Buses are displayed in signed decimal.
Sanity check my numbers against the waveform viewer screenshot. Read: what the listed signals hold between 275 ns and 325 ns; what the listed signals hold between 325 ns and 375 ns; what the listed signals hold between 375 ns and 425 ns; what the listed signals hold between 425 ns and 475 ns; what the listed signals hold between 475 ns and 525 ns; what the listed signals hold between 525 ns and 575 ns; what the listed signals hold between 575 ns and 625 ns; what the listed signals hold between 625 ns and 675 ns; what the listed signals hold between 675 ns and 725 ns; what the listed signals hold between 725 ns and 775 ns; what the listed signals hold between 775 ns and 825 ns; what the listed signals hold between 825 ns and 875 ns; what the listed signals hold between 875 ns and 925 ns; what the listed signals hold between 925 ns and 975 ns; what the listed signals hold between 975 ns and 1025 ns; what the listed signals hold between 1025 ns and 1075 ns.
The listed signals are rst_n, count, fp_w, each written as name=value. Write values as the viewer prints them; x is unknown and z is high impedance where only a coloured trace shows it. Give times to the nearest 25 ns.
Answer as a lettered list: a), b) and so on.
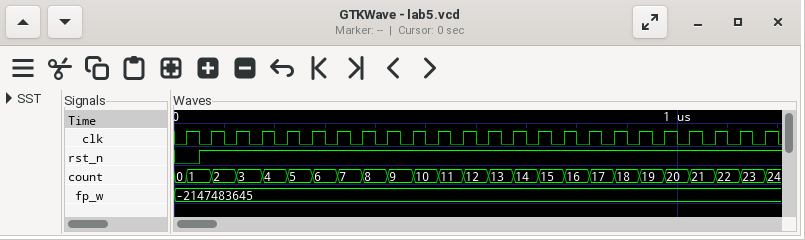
a) rst_n=1, count=6, fp_w=-2147483645
b) rst_n=1, count=7, fp_w=-2147483645
c) rst_n=1, count=8, fp_w=-2147483645
d) rst_n=1, count=9, fp_w=-2147483645
e) rst_n=1, count=10, fp_w=-2147483645
f) rst_n=1, count=11, fp_w=-2147483645
g) rst_n=1, count=12, fp_w=-2147483645
h) rst_n=1, count=13, fp_w=-2147483645
i) rst_n=1, count=14, fp_w=-2147483645
j) rst_n=1, count=15, fp_w=-2147483645
k) rst_n=1, count=16, fp_w=-2147483645
l) rst_n=1, count=17, fp_w=-2147483645
m) rst_n=1, count=18, fp_w=-2147483645
n) rst_n=1, count=19, fp_w=-2147483645
o) rst_n=1, count=20, fp_w=-2147483645
p) rst_n=1, count=21, fp_w=-2147483645
